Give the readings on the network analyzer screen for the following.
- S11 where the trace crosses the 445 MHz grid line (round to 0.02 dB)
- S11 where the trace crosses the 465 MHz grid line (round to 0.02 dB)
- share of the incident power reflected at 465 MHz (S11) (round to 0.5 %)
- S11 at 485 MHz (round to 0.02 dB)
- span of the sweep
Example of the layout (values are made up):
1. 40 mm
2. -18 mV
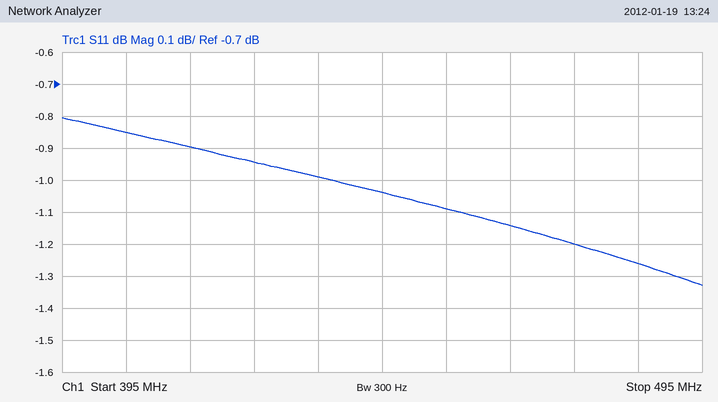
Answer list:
1. -1.04 dB
2. -1.14 dB
3. 77.0 %
4. -1.26 dB
5. 100 MHz
